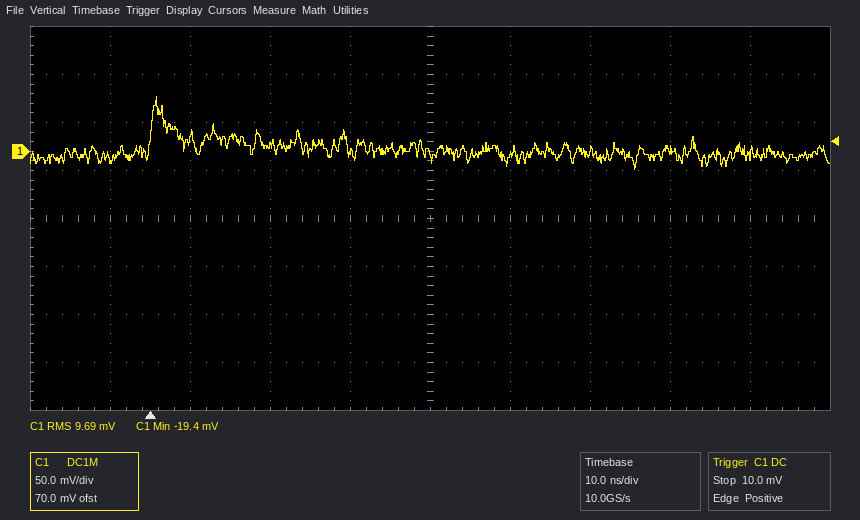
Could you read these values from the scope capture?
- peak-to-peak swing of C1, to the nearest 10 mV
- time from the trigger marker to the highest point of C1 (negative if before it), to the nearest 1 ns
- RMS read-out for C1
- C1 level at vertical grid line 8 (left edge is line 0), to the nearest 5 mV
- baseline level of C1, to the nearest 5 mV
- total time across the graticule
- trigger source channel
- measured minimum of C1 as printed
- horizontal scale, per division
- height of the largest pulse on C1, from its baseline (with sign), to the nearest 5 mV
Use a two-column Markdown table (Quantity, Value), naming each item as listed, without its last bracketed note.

| Quantity | Value |
|---|---|
| peak-to-peak swing of C1, to the nearest 10 mV | 80 mV |
| time from the trigger marker to the highest point of C1 (negative if before it), to the nearest 1 ns | +1 ns |
| RMS read-out for C1 | 9.69 mV |
| C1 level at vertical grid line 8 (left edge is line 0), to the nearest 5 mV | 0 mV |
| baseline level of C1, to the nearest 5 mV | 0 mV |
| total time across the graticule | 100 ns |
| trigger source channel | C1 |
| measured minimum of C1 as printed | -19.4 mV |
| horizontal scale, per division | 10 ns |
| height of the largest pulse on C1, from its baseline (with sign), to the nearest 5 mV | +60 mV |
